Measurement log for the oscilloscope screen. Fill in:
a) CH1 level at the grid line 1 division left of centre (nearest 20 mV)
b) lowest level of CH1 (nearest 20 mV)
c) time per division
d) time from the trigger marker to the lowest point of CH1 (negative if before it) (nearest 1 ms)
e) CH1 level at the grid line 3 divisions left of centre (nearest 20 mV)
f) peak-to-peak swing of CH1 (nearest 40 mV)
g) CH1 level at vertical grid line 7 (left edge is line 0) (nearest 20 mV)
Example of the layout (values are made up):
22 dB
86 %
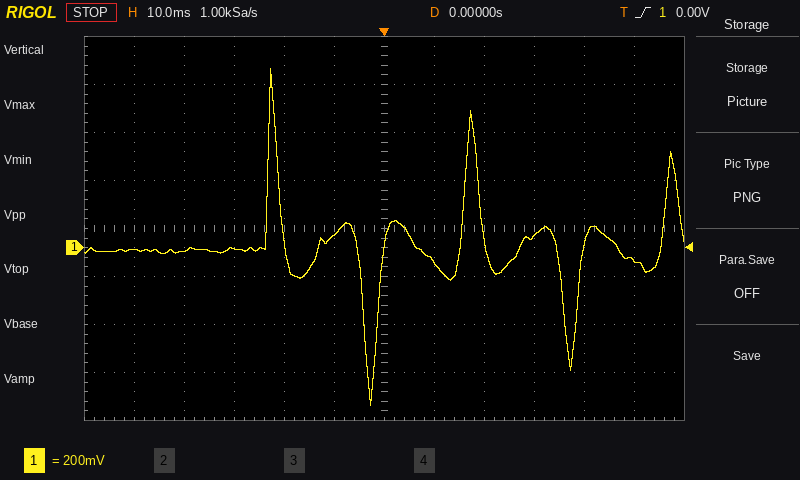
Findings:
60 mV
-660 mV
10 ms
-3 ms
0 mV
1.40 V
-60 mV
